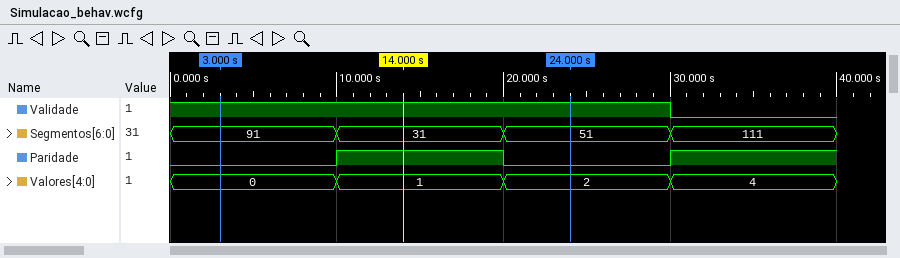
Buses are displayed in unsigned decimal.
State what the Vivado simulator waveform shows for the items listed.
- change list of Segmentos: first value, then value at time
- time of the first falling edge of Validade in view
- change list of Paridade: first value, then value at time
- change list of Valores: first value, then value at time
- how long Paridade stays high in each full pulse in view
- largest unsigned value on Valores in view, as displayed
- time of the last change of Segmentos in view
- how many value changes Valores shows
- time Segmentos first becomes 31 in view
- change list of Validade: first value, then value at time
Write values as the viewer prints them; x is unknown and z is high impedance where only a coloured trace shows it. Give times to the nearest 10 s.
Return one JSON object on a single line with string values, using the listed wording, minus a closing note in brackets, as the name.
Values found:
{"change list of Segmentos: first value, then value at time": "91, 31 at 10 s, 51 at 20 s, 111 at 30 s", "time of the first falling edge of Validade in view": "30 s", "change list of Paridade: first value, then value at time": "0, 1 at 10 s, 0 at 20 s, 1 at 30 s", "change list of Valores: first value, then value at time": "0, 1 at 10 s, 2 at 20 s, 4 at 30 s", "how long Paridade stays high in each full pulse in view": "10 s", "largest unsigned value on Valores in view, as displayed": "4", "time of the last change of Segmentos in view": "30 s", "how many value changes Valores shows": "3", "time Segmentos first becomes 31 in view": "10 s", "change list of Validade: first value, then value at time": "1, 0 at 30 s"}
